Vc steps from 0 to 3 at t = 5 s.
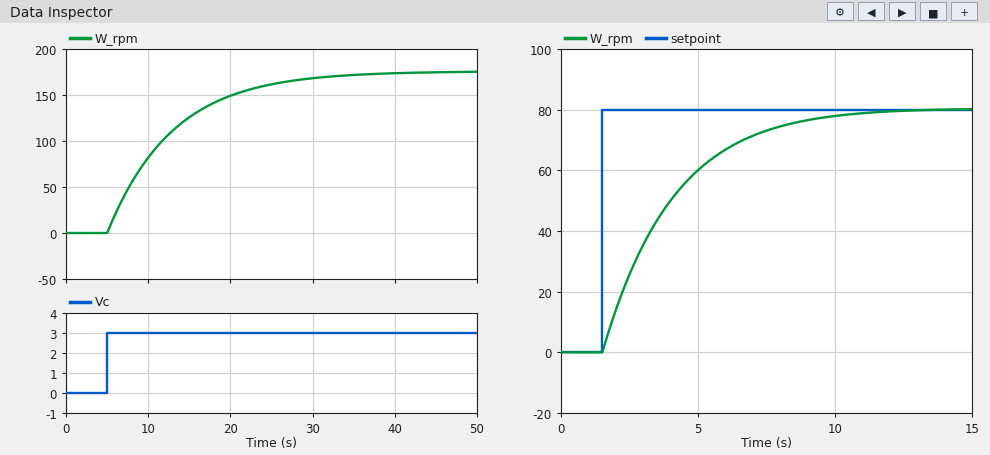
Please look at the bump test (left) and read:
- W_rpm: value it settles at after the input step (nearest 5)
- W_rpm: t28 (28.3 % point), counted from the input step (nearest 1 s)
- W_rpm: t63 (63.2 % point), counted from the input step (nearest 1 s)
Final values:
175
3 s
8 s
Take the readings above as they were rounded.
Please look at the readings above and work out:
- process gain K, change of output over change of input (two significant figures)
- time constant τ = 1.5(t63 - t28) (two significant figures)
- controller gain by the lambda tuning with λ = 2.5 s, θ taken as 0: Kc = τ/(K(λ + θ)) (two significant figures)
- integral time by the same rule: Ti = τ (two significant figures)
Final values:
58
7.5 s
0.052
7.5 s
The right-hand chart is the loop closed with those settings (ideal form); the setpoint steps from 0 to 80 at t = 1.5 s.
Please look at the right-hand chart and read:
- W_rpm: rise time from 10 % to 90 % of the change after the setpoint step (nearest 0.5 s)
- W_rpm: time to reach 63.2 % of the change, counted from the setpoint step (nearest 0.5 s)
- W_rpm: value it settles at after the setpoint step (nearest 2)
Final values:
5.5 s
2.5 s
80
